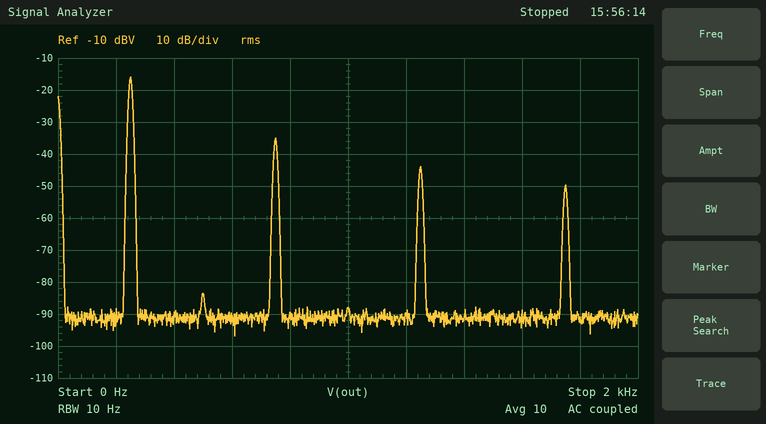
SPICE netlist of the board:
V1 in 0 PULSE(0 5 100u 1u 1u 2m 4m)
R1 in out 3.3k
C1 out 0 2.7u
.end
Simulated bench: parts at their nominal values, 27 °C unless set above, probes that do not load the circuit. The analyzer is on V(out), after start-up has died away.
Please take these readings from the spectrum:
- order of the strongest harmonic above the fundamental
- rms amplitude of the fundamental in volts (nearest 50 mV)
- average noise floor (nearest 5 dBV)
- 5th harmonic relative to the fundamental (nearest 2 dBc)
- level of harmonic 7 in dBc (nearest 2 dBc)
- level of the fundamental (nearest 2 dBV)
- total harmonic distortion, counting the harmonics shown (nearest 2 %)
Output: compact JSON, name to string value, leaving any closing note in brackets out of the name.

{"order of the strongest harmonic above the fundamental": "3", "rms amplitude of the fundamental in volts": "150 mV", "average noise floor": "-90 dBV", "5th harmonic relative to the fundamental": "-28 dBc", "level of harmonic 7 in dBc": "-34 dBc", "level of the fundamental": "-16 dBV", "total harmonic distortion, counting the harmonics shown": "12 %"}
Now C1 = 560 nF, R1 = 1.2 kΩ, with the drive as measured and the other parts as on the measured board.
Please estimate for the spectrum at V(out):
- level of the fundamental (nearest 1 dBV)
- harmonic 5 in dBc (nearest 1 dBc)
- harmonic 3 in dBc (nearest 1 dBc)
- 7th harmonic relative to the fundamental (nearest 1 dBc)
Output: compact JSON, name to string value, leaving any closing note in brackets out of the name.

{"level of the fundamental": "4 dBV", "harmonic 5 in dBc": "-25 dBc", "harmonic 3 in dBc": "-17 dBc", "7th harmonic relative to the fundamental": "-31 dBc"}
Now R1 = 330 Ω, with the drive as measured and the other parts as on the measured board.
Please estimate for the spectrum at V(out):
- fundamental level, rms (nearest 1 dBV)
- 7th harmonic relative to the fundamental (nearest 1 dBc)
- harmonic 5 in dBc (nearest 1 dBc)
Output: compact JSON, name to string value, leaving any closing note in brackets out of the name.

{"fundamental level, rms": "2 dBV", "7th harmonic relative to the fundamental": "-32 dBc", "harmonic 5 in dBc": "-26 dBc"}
